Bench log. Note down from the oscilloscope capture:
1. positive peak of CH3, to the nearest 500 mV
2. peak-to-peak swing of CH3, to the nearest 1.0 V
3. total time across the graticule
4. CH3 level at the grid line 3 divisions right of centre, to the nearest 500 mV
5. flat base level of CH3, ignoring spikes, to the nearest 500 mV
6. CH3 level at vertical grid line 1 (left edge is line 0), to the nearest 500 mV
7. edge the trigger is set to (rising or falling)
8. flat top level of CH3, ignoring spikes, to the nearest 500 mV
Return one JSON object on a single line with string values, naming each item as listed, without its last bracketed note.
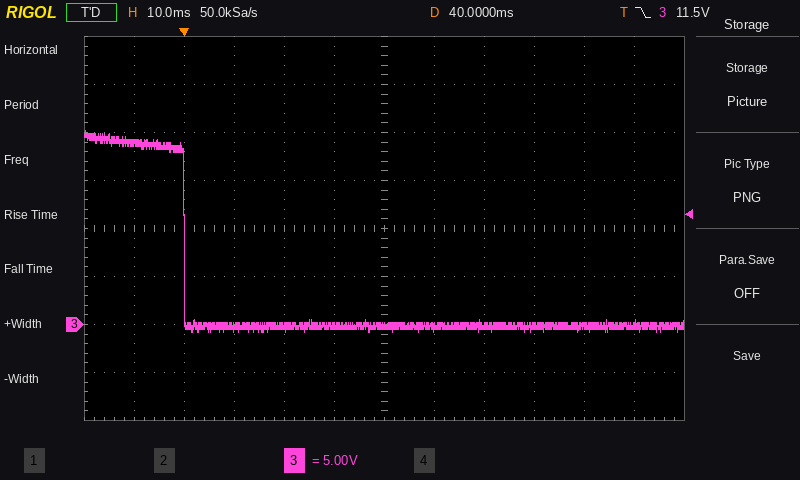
{"positive peak of CH3, to the nearest 500 mV": "20.0 V", "peak-to-peak swing of CH3, to the nearest 1.0 V": "21.0 V", "total time across the graticule": "120 ms", "CH3 level at the grid line 3 divisions right of centre, to the nearest 500 mV": "0.0 V", "flat base level of CH3, ignoring spikes, to the nearest 500 mV": "0.0 V", "CH3 level at vertical grid line 1 (left edge is line 0), to the nearest 500 mV": "19.0 V", "edge the trigger is set to": "falling", "flat top level of CH3, ignoring spikes, to the nearest 500 mV": "19.0 V"}
